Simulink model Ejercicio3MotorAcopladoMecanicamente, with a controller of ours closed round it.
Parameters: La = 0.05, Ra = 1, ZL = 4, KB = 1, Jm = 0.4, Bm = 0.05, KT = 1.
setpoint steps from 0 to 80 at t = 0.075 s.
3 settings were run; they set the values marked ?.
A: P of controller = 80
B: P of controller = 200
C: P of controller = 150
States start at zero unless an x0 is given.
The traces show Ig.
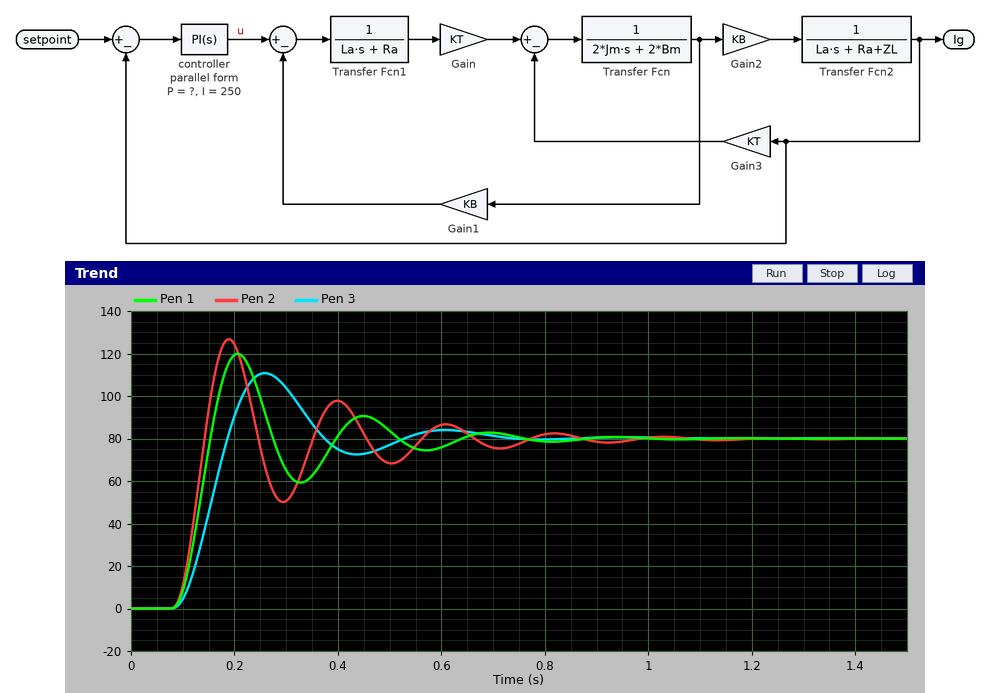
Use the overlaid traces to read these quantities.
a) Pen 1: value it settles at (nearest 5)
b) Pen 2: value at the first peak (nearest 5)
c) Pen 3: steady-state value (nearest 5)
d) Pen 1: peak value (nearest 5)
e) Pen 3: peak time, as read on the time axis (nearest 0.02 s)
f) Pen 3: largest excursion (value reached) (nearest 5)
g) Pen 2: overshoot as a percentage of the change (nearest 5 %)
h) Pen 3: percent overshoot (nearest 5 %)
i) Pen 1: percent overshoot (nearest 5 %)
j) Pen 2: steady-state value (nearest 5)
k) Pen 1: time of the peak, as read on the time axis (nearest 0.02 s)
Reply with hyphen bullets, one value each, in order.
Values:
- 80
- 125
- 80
- 120
- 0.26 s
- 110
- 60 %
- 40 %
- 50 %
- 80
- 0.20 s
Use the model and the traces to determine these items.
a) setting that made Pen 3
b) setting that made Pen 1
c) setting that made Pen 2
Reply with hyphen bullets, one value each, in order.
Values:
- A
- C
- B
